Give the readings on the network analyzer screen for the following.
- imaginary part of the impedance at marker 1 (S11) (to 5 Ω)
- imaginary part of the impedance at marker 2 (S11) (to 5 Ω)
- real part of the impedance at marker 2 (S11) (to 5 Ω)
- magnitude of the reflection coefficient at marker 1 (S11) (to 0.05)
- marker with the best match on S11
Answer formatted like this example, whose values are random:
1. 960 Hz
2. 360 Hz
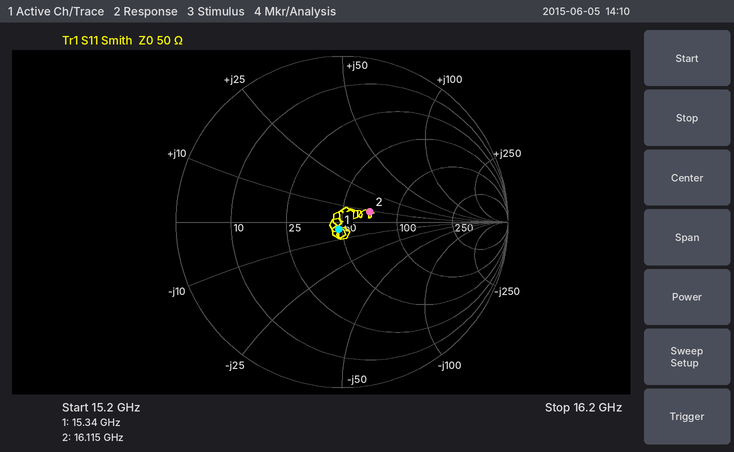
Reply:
1. -5 Ω
2. +10 Ω
3. 70 Ω
4. 0.05
5. marker 1
